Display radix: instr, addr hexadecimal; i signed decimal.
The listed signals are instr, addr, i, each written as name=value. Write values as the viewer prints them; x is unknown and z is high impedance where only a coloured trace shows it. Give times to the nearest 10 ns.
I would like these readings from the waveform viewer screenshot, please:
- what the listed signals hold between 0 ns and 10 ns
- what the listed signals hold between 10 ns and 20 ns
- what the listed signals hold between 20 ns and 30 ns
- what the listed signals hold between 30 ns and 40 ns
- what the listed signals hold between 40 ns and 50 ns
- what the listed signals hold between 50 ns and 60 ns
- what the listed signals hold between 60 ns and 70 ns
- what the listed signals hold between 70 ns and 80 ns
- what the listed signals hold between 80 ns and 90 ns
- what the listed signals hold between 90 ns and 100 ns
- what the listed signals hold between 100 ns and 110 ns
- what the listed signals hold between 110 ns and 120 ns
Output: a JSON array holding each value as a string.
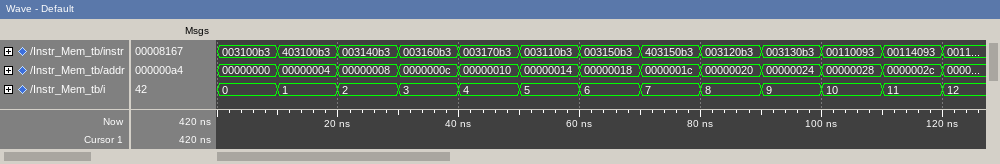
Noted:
["instr=003100b3, addr=00000000, i=0", "instr=403100b3, addr=00000004, i=1", "instr=003140b3, addr=00000008, i=2", "instr=003160b3, addr=0000000c, i=3", "instr=003170b3, addr=00000010, i=4", "instr=003110b3, addr=00000014, i=5", "instr=003150b3, addr=00000018, i=6", "instr=403150b3, addr=0000001c, i=7", "instr=003120b3, addr=00000020, i=8", "instr=003130b3, addr=00000024, i=9", "instr=00110093, addr=00000028, i=10", "instr=00114093, addr=0000002c, i=11"]
